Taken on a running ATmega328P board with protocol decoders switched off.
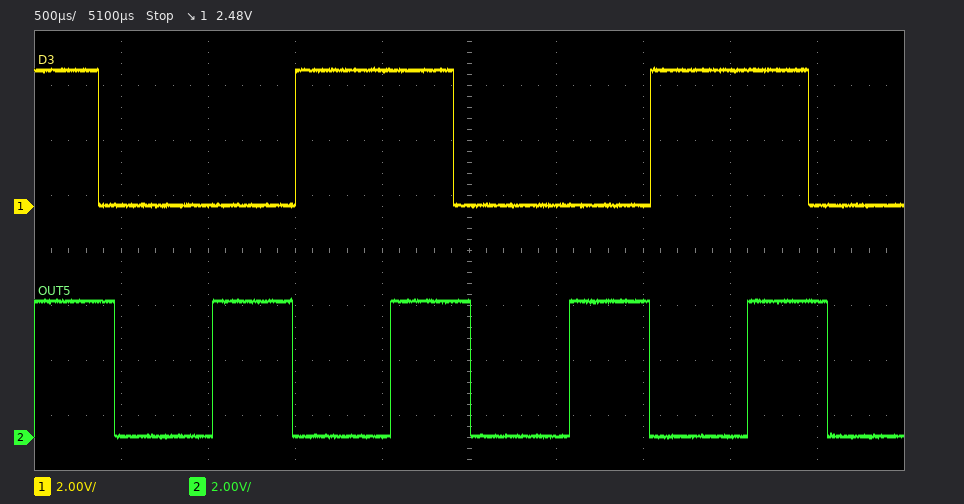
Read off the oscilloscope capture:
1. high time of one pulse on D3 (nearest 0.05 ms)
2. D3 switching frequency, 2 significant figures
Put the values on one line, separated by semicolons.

0.90 ms; 490 Hz
